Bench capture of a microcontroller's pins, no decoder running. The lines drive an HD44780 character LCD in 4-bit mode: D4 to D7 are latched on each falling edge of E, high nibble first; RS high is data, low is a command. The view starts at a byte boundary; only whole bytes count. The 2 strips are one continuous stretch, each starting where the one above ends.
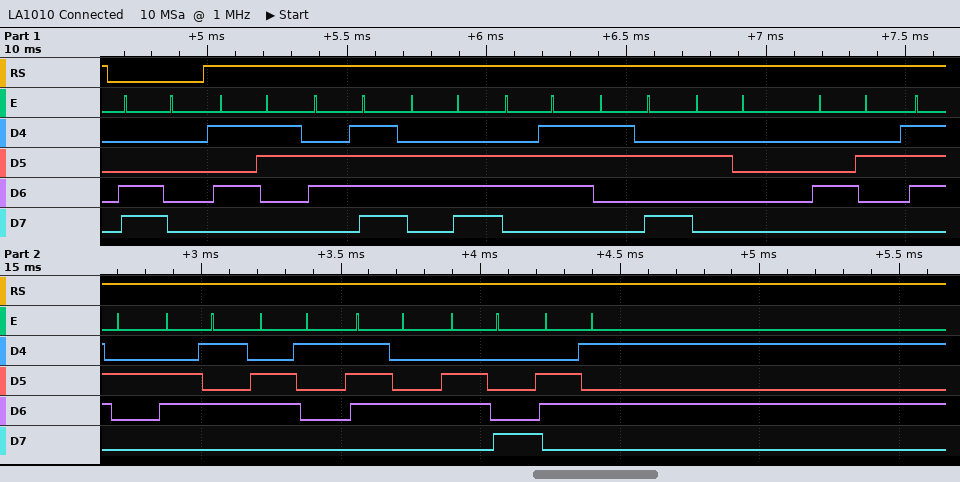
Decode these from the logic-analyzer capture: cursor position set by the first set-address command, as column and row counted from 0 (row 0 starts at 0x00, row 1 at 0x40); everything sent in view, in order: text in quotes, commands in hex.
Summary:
column 0, row 1
0xC0 "Song: Breathe"
